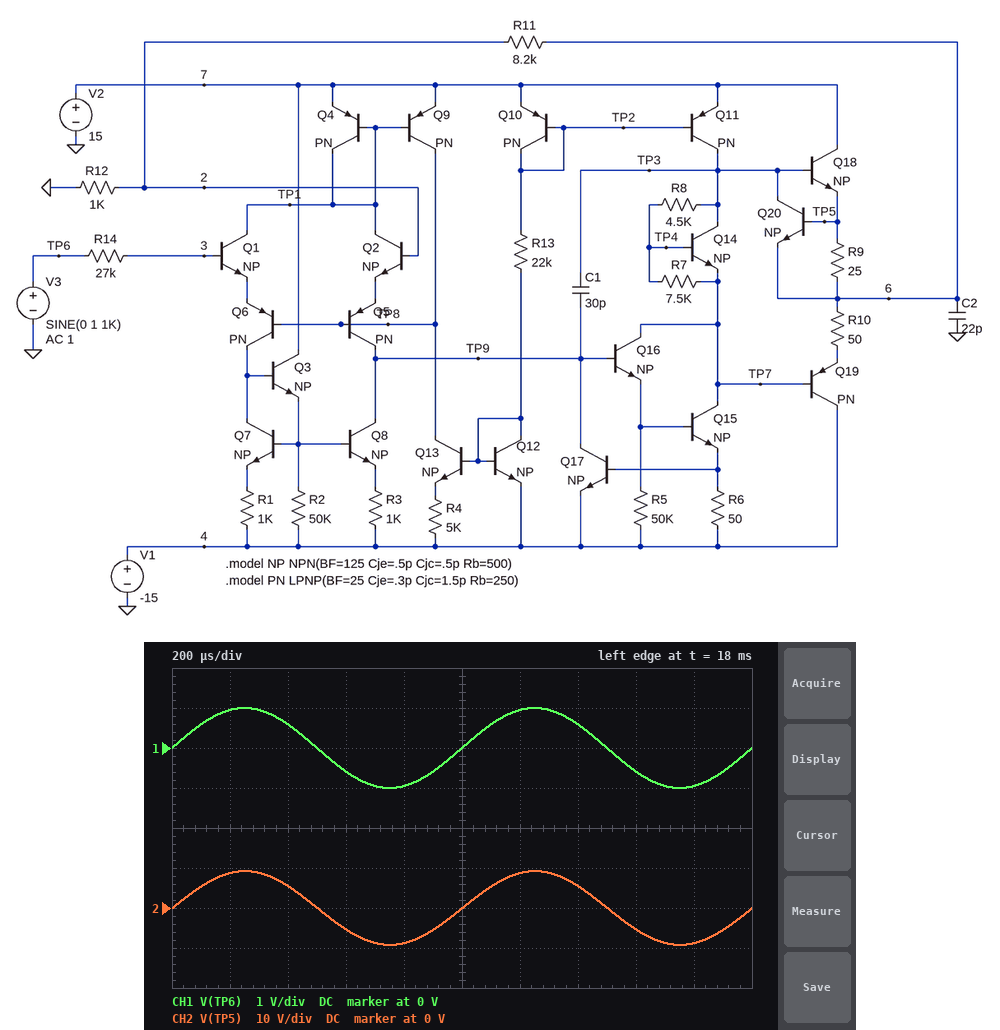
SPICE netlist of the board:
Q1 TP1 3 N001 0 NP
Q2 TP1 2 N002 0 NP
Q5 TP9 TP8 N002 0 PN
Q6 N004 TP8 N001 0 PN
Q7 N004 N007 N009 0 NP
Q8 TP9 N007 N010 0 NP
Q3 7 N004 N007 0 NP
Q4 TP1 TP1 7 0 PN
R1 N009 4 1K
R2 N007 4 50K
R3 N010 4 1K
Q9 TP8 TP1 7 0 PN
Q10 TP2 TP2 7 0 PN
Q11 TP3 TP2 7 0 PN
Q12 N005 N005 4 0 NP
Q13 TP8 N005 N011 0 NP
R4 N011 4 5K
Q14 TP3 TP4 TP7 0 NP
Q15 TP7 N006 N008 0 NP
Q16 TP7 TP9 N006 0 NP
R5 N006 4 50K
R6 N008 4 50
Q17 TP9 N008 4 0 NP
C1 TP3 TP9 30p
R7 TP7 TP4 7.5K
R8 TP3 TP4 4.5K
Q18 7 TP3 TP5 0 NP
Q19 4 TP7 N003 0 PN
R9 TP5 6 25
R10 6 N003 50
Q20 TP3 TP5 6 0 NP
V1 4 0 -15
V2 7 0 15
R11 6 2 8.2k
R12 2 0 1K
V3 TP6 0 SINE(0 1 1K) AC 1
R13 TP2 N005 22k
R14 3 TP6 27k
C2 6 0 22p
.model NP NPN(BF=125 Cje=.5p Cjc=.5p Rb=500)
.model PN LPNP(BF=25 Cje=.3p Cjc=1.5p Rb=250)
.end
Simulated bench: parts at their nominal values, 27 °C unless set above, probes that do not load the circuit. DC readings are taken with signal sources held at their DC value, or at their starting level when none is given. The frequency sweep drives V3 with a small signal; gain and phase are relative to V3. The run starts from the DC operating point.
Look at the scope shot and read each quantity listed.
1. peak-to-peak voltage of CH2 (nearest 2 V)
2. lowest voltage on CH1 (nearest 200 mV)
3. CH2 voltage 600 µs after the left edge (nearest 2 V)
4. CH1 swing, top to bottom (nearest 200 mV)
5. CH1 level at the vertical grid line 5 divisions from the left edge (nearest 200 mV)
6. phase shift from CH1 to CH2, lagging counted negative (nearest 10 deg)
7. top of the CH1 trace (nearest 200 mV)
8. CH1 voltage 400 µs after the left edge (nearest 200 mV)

18 V
-1.0 V
-6 V
2.0 V
0 V
0 deg
1.0 V
600 mV
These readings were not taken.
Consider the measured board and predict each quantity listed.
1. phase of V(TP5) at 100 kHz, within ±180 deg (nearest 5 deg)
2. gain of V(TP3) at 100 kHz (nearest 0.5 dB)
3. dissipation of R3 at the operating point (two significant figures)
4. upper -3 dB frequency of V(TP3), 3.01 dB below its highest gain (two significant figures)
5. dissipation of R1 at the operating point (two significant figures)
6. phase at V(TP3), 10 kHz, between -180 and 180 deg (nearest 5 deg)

-45 deg
18.0 dB
120 nW
100 kHz
120 nW
-5 deg
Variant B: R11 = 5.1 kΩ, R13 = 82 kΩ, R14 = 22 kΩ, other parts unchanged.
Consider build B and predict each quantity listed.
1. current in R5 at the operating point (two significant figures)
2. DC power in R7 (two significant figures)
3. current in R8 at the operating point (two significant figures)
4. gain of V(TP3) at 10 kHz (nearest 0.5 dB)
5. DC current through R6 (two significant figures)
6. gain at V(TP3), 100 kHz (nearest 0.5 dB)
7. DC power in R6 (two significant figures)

15 µA
72 µW
100 µA
25.0 dB
310 µA
17.5 dB
4.7 µW
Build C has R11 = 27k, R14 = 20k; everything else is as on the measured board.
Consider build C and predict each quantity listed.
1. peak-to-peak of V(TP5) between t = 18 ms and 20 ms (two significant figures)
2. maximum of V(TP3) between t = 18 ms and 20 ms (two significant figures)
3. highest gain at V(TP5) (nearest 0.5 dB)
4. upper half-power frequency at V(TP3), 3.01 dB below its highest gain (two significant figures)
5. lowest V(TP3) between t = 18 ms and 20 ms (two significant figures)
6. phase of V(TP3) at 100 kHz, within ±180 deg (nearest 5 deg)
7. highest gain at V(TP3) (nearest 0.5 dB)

28 V
15 V
29.0 dB
37 kHz
-13 V
-70 deg
29.5 dB
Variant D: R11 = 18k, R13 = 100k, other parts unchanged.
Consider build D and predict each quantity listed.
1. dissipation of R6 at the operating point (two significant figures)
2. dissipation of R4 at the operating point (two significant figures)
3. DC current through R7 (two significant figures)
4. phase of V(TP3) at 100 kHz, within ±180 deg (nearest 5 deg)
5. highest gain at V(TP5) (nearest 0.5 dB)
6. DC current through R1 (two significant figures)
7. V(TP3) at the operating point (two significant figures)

3.1 µW
1.2 µW
97 µA
-75 deg
25.5 dB
7.6 µA
540 mV
